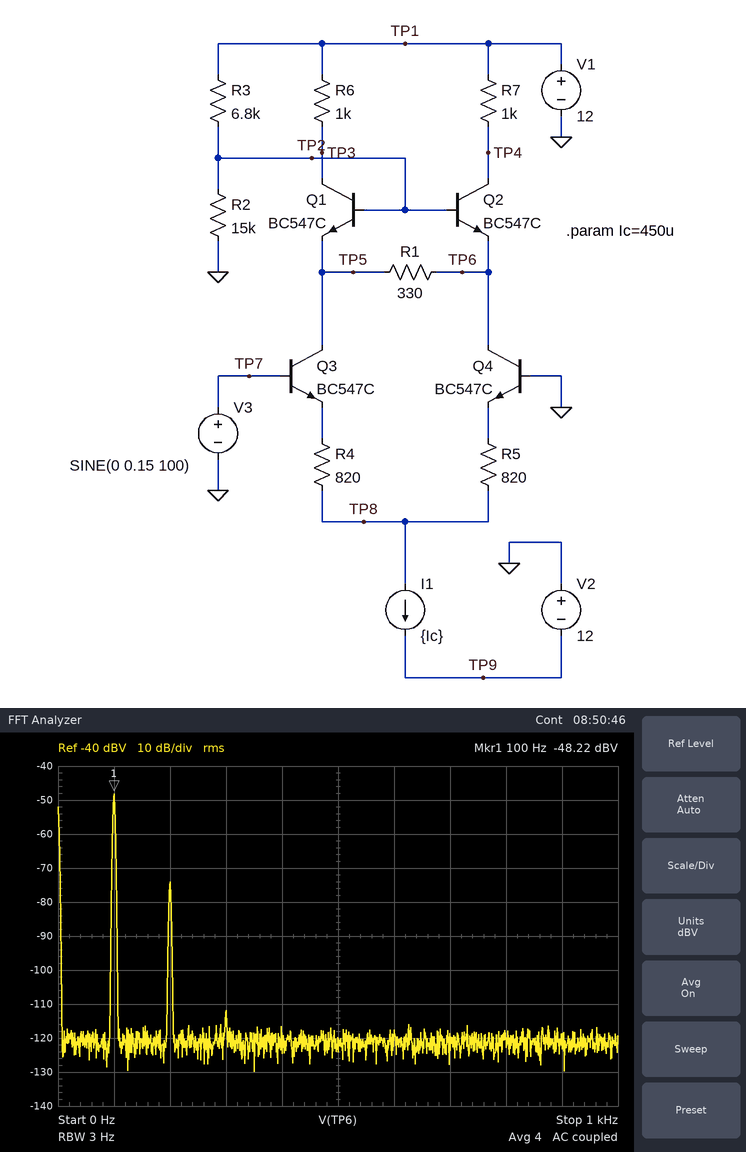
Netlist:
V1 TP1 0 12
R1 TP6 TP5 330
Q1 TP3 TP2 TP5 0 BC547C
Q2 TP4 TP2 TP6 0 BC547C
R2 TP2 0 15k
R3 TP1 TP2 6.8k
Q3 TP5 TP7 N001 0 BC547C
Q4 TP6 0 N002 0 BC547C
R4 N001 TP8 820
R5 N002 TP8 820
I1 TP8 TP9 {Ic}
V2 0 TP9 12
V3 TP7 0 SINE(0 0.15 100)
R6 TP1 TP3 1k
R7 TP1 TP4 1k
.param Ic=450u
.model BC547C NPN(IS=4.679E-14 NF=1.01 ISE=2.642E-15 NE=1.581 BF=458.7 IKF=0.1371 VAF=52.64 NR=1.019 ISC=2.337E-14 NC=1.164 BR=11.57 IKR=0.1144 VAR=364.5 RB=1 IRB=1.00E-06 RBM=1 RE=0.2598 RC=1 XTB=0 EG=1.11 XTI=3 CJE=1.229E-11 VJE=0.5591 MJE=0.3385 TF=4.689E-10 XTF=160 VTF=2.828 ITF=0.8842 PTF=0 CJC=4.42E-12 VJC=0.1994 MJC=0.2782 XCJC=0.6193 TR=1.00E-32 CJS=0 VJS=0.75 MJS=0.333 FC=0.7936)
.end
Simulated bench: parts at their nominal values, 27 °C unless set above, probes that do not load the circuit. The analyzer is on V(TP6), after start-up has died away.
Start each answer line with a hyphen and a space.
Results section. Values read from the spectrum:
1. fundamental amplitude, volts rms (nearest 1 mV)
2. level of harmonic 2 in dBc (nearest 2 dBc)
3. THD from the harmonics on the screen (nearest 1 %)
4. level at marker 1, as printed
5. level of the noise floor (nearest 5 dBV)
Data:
- 4 mV
- -26 dBc
- 5 %
- -48.22 dBV
- -120 dBV
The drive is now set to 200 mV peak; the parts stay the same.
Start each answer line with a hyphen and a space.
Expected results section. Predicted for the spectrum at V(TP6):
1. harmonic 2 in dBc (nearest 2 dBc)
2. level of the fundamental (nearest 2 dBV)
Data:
- -24 dBc
- -46 dBV
